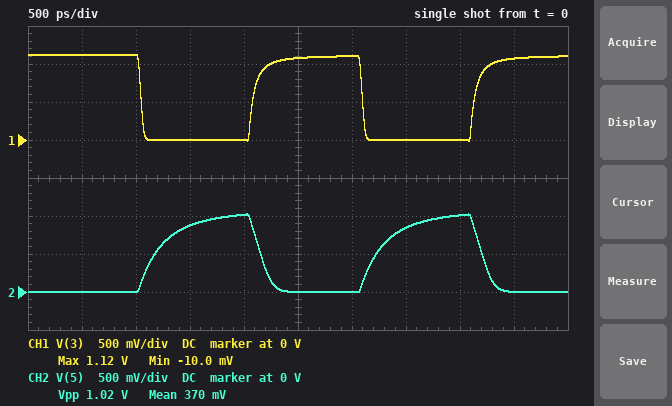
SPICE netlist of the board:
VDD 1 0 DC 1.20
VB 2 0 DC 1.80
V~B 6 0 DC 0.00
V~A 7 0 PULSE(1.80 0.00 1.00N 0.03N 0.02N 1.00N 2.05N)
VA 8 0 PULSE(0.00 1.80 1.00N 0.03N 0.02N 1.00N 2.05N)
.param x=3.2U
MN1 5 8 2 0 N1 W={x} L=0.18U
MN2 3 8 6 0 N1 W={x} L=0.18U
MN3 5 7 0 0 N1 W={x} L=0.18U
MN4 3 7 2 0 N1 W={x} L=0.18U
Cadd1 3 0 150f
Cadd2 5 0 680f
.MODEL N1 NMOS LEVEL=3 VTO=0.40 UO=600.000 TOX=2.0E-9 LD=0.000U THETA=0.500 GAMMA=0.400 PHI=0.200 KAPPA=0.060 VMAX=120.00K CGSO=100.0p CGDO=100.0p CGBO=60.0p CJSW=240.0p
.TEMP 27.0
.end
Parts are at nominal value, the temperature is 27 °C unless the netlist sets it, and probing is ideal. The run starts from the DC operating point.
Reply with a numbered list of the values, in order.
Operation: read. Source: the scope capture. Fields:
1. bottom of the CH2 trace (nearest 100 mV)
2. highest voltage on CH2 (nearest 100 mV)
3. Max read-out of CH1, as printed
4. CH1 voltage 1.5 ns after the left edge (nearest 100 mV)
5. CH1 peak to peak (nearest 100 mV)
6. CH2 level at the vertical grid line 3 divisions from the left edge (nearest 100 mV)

1. 0 V
2. 1.0 V
3. 1.12 V
4. 0 V
5. 1.1 V
6. 900 mV
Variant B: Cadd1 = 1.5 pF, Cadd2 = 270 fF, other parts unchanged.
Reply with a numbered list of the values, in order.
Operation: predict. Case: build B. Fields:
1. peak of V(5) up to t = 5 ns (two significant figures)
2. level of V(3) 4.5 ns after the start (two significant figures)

1. 1.1 V
2. 560 mV
